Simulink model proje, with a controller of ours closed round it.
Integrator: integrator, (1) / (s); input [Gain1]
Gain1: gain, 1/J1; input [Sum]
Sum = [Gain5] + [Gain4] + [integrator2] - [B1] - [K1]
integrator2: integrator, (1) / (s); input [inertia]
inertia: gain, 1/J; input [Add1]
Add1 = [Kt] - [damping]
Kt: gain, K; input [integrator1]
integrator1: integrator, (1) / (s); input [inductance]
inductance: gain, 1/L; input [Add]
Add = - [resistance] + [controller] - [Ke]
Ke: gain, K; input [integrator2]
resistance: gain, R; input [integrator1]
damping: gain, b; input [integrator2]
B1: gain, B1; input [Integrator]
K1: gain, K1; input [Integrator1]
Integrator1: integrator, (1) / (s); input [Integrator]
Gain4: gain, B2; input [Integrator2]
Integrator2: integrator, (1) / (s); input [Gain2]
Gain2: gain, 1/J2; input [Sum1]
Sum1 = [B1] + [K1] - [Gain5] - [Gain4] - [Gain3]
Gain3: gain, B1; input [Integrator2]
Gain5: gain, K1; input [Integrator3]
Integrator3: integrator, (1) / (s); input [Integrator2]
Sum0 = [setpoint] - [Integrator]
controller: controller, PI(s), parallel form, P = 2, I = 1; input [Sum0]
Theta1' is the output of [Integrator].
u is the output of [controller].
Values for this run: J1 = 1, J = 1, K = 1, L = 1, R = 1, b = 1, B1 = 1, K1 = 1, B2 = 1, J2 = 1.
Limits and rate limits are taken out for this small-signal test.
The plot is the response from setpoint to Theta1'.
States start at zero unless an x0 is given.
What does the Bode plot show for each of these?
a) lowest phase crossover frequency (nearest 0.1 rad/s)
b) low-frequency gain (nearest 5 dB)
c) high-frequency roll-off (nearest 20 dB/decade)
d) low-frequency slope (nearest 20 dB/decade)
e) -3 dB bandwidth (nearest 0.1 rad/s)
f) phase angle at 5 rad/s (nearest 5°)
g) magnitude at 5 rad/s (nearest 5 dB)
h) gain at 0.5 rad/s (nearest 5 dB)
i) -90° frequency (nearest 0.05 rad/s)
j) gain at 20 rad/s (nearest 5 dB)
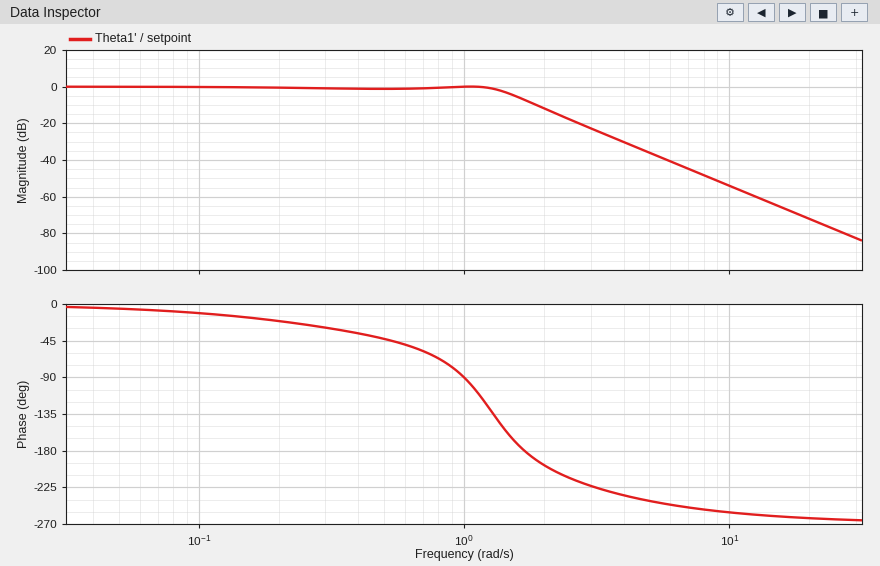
1.7 rad/s
0 dB
-60 dB/decade
0 dB/decade
1.4 rad/s
-240°
-35 dB
0 dB
1.00 rad/s
-70 dB
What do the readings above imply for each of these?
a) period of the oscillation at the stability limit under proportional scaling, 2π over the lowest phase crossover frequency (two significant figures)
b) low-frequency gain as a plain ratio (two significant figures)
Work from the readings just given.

3.7 s
1.0
